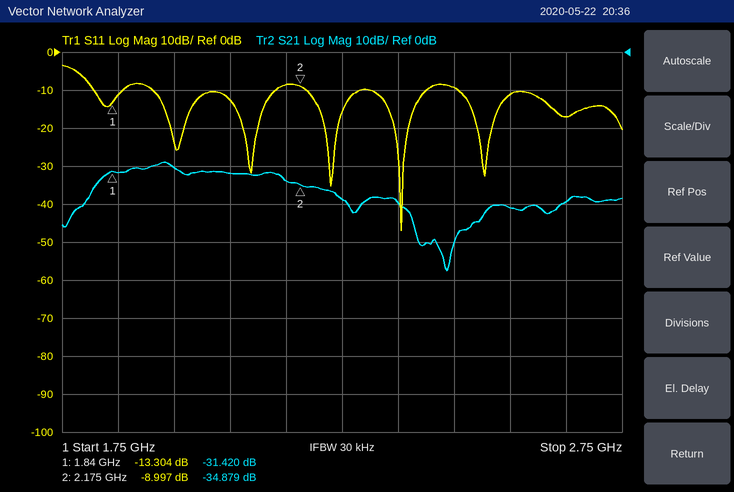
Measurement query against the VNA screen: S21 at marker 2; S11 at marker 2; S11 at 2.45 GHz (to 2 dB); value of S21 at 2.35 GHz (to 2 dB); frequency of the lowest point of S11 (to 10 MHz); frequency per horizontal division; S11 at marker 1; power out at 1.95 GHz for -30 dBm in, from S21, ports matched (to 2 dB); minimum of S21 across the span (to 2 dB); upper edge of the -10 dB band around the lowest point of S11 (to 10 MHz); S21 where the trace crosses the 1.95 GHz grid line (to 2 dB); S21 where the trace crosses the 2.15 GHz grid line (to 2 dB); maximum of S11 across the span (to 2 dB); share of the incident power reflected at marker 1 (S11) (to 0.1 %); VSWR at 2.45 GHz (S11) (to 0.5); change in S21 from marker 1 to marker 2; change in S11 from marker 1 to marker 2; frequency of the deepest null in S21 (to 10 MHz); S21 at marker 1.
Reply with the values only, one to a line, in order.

-34.879 dB
-8.997 dB
-10 dB
-40 dB
2.36 GHz
100 MHz
-13.304 dB
-60 dBm
-58 dB
2.40 GHz
-30 dB
-34 dB
-4 dB
4.7 %
2.0
-3.459 dB
4.307 dB
2.44 GHz
-31.420 dB
